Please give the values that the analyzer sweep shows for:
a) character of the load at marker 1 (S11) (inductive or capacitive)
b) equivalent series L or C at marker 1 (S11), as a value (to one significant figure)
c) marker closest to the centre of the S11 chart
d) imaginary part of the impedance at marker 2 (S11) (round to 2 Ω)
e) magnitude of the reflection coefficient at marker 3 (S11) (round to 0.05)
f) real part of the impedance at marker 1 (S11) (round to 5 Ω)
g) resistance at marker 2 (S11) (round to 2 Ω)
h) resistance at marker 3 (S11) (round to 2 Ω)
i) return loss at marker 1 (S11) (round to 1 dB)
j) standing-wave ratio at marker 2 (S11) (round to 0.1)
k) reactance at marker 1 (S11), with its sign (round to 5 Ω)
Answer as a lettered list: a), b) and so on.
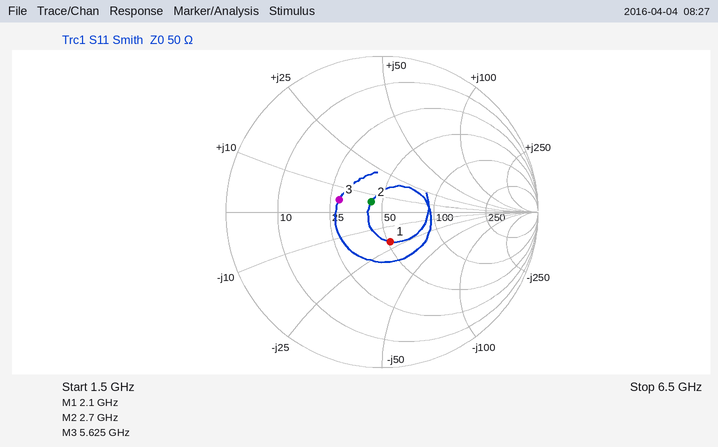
a) capacitive
b) 4 pF
c) marker 2
d) +6 Ω
e) 0.30
f) 50 Ω
g) 44 Ω
h) 28 Ω
i) 14 dB
j) 1.2
k) -20 Ω
